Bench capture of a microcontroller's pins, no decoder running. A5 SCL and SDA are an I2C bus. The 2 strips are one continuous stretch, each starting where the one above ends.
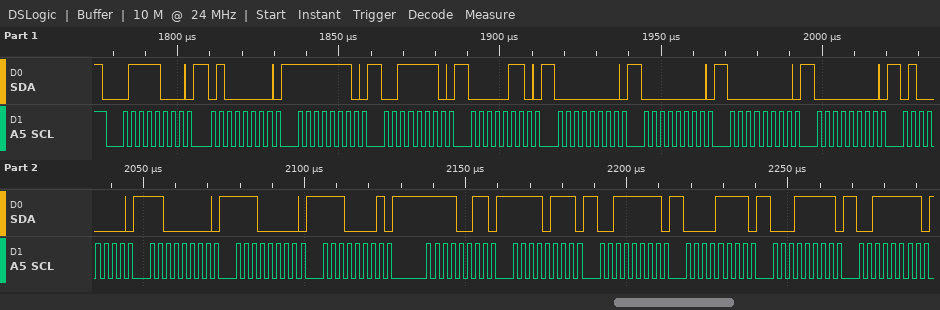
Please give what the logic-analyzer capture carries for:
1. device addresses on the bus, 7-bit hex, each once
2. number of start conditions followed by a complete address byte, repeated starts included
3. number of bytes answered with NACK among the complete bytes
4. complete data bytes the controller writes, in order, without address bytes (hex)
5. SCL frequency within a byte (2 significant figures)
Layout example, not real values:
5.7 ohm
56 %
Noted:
0x3C
1
0
40 FE 3E 06 00 00 00 00 40 C0 E0 E1 F3 F7 3F 0F 1F 3F
400 kHz
